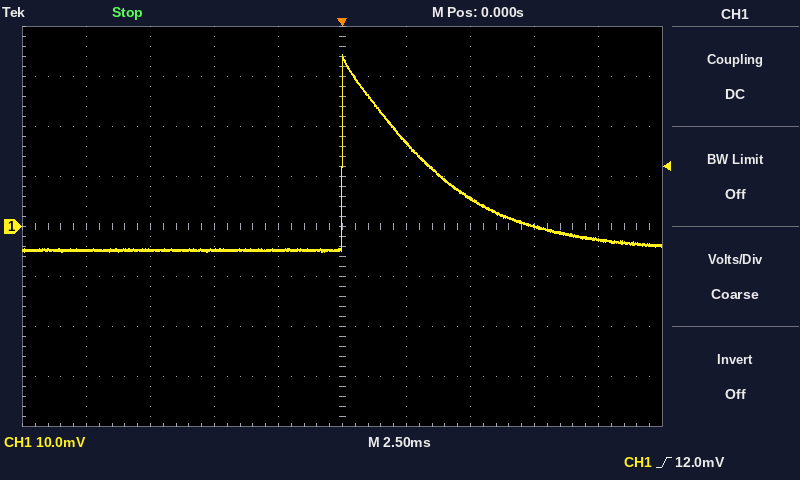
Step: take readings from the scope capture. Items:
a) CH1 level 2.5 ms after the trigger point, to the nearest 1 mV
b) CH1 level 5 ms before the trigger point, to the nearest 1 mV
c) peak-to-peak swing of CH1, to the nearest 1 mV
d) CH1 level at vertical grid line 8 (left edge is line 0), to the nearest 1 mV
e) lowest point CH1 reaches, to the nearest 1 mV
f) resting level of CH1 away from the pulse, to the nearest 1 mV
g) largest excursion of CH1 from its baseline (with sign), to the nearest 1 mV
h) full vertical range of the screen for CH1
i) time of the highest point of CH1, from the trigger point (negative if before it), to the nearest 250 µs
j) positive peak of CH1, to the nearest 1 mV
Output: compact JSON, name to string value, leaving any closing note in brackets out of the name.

{"CH1 level 2.5 ms after the trigger point, to the nearest 1 mV": "17 mV", "CH1 level 5 ms before the trigger point, to the nearest 1 mV": "-5 mV", "peak-to-peak swing of CH1, to the nearest 1 mV": "39 mV", "CH1 level at vertical grid line 8 (left edge is line 0), to the nearest 1 mV": "0 mV", "lowest point CH1 reaches, to the nearest 1 mV": "-5 mV", "resting level of CH1 away from the pulse, to the nearest 1 mV": "-5 mV", "largest excursion of CH1 from its baseline (with sign), to the nearest 1 mV": "+39 mV", "full vertical range of the screen for CH1": "80 mV", "time of the highest point of CH1, from the trigger point (negative if before it), to the nearest 250 µs": "0.00 ms", "positive peak of CH1, to the nearest 1 mV": "34 mV"}
